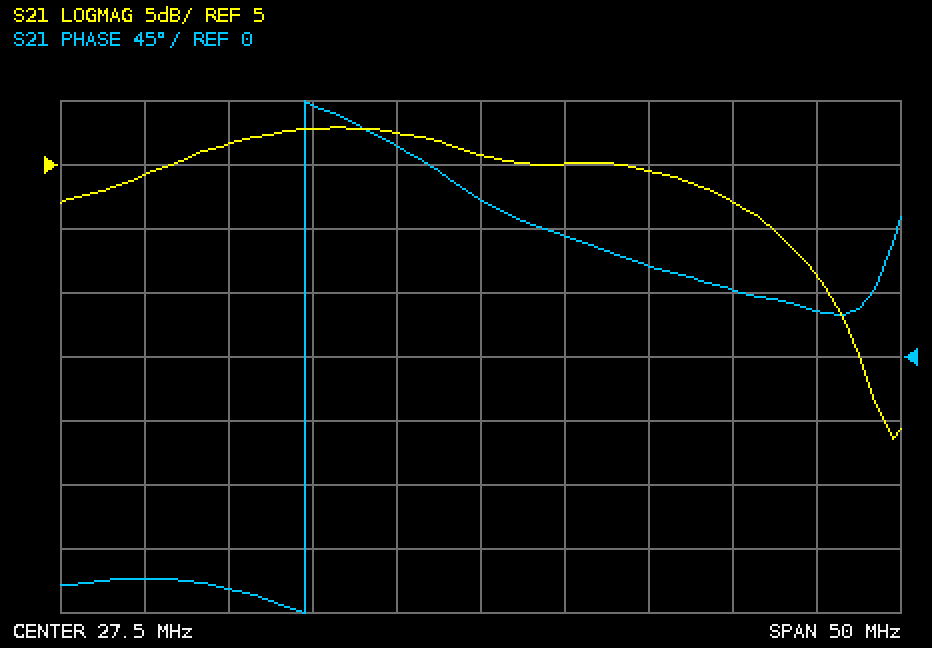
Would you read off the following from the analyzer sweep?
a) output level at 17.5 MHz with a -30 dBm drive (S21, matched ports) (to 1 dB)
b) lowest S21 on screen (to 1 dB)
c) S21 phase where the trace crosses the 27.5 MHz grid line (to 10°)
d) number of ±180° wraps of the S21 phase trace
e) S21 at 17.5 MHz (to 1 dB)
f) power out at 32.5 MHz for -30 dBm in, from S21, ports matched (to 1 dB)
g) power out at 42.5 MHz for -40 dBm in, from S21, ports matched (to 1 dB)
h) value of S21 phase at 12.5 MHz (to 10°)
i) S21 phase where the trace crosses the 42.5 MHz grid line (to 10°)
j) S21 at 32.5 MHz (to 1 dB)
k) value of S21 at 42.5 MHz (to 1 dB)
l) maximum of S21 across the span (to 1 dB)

-22 dBm
-16 dB
110°
1
8 dB
-25 dBm
-38 dBm
-160°
50°
5 dB
2 dB
8 dB
